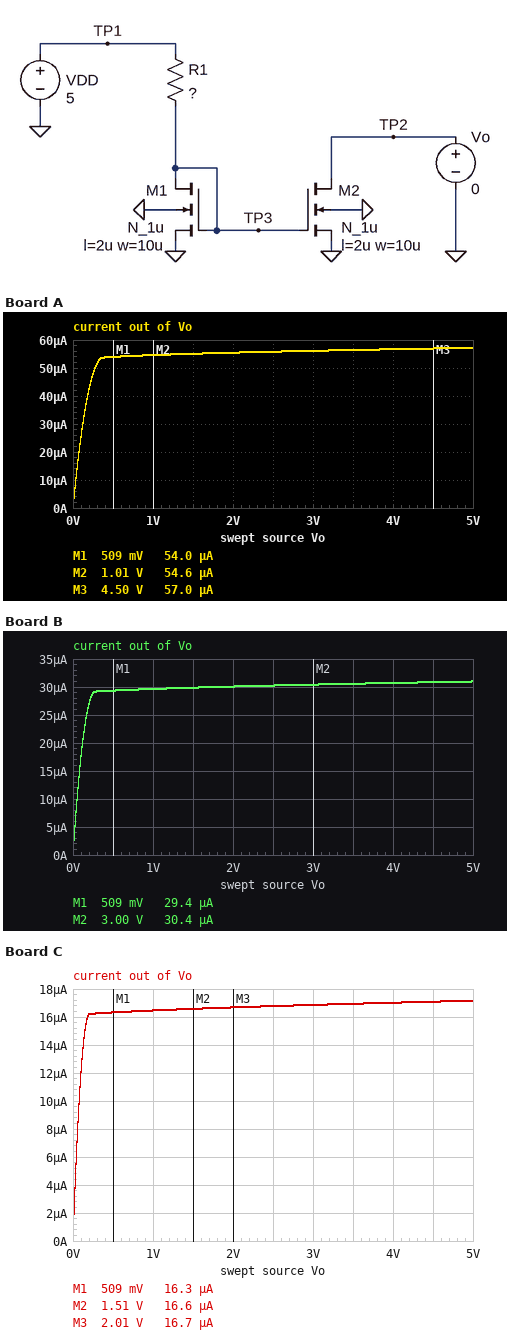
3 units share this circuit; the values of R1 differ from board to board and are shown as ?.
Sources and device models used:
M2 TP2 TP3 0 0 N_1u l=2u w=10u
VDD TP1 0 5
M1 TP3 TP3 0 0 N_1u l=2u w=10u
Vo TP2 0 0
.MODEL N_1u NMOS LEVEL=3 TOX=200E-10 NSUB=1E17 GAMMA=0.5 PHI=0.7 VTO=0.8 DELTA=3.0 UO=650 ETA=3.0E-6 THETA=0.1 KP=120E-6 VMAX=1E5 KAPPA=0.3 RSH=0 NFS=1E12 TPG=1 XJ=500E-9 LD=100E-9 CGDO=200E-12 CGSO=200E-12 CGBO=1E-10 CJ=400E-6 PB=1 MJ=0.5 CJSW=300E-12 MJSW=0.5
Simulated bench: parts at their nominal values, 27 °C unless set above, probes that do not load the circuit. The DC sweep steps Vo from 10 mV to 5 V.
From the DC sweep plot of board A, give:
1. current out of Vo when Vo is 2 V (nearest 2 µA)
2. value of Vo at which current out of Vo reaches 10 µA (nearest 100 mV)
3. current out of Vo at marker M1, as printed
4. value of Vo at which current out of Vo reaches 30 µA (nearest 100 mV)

56 µA
0 V
54.0 µA
100 mV
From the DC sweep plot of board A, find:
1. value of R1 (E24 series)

68 kΩ
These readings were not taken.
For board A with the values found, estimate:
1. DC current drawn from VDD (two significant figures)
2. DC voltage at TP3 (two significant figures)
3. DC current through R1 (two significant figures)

55 µA
1.3 V
55 µA
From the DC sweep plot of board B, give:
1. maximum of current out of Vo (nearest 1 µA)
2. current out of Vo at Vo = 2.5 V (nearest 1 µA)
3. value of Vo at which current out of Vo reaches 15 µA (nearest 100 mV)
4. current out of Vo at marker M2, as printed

31 µA
30 µA
100 mV
30.4 µA
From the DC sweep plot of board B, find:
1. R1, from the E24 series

130 kΩ
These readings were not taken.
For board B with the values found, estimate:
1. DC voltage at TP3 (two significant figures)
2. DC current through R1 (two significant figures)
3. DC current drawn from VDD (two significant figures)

1.1 V
30 µA
30 µA
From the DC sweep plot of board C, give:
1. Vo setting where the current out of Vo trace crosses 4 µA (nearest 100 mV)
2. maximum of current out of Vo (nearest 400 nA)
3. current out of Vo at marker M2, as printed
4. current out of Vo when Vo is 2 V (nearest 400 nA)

0 V
17.2 µA
16.6 µA
16.8 µA
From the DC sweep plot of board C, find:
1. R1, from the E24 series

240 kΩ
